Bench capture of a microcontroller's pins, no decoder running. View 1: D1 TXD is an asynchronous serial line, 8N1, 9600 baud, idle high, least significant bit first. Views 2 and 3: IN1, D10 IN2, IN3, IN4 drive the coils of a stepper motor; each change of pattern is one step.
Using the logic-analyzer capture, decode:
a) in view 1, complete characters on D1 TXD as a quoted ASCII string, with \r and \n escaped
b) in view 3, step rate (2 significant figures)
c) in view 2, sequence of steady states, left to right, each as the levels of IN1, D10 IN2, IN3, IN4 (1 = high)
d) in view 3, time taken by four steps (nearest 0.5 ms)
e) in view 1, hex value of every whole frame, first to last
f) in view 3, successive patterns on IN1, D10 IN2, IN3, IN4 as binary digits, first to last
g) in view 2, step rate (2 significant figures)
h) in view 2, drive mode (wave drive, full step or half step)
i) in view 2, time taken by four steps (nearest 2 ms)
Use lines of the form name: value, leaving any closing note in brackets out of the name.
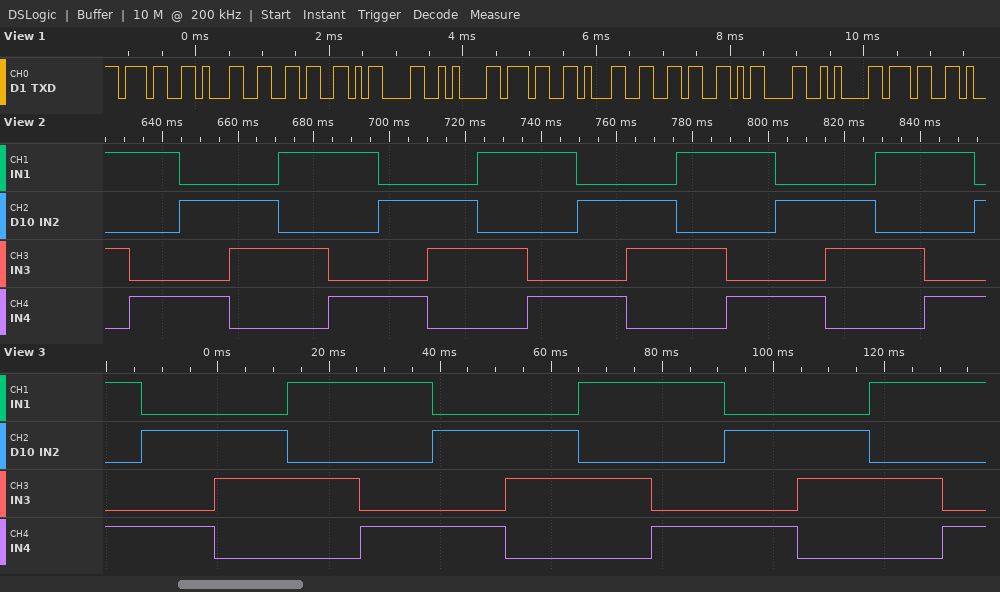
in view 1, complete characters on D1 TXD as a quoted ASCII string, with \r and \n escaped: "716\r\n716\r\n7"
in view 3, step rate: 76 steps/s
in view 2, sequence of steady states, left to right, each as the levels of IN1, D10 IN2, IN3, IN4: 1010 1001 0101 0110 1010 1001 0101 0110 1010 1001 0101 0110 1010 1001 0101 0110 1010 1001 0101
in view 3, time taken by four steps: 52.5 ms
in view 1, hex value of every whole frame, first to last: 37 31 36 0D 0A 37 31 36 0D 0A 37
in view 3, successive patterns on IN1, D10 IN2, IN3, IN4 as binary digits, first to last: 1001 0101 0110 1010 1001 0101 0110 1010 1001 0101 0110 1010 1001
in view 2, step rate: 76 steps/s
in view 2, drive mode: full step
in view 2, time taken by four steps: 52 ms
